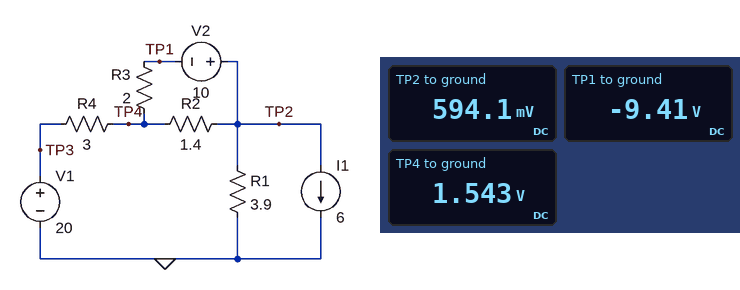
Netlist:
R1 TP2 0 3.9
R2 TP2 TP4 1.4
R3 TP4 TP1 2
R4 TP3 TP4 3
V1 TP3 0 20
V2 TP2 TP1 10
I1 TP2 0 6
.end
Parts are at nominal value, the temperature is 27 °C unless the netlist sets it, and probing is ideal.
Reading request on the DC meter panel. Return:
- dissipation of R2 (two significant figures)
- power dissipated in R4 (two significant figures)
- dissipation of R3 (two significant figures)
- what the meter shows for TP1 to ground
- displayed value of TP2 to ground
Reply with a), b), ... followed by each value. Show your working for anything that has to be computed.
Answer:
a) (1.543 V - 594.1 mV)^2 / 1.4 Ω = 640 mW
b) (20 V - 1.543 V)^2 / 3 Ω = 110 W
c) (1.543 V - (-9.41 V))^2 / 2 Ω = 60 W
d) -9.41 V
e) 594.1 mV
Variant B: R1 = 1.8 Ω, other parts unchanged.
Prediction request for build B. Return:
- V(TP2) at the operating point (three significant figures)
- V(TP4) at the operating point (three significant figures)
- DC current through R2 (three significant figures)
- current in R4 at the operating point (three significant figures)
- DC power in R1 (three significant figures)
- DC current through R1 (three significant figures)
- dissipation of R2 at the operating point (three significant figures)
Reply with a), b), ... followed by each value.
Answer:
a) 377 mV
b) 1.37 V
c) 711 mA
d) 6.21 A
e) 78.8 mW
f) 209 mA
g) 708 mW
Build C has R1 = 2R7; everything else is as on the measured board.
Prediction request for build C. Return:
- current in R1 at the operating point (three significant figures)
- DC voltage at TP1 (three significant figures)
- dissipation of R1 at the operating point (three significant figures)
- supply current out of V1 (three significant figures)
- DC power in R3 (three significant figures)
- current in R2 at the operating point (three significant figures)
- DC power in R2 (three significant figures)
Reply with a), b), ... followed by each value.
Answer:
a) 180 mA
b) -9.51 V
c) 87.8 mW
d) 6.18 A
e) 60.2 W
f) 694 mA
g) 675 mW
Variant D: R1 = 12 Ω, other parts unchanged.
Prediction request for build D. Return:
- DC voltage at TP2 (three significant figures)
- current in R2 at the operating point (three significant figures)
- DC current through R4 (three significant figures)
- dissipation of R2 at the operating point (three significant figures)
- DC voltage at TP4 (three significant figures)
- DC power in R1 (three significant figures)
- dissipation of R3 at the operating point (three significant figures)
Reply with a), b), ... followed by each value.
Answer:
a) 892 mV
b) 632 mA
c) 6.07 A
d) 559 mW
e) 1.78 V
f) 66.3 mW
g) 59.2 W
